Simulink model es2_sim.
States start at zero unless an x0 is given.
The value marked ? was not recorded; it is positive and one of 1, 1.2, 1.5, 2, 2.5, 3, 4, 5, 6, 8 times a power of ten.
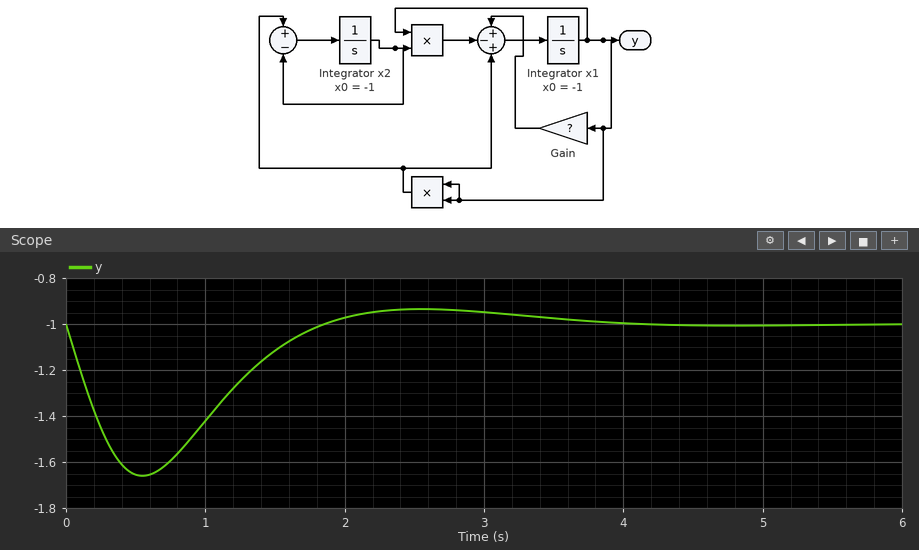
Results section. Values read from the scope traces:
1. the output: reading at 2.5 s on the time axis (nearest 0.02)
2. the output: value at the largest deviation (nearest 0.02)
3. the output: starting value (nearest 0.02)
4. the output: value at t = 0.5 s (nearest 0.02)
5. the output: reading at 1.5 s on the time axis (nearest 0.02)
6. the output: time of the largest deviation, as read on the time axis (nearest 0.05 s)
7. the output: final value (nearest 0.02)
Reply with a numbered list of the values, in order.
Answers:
1. -0.94
2. -1.66
3. -1.00
4. -1.66
5. -1.12
6. 0.55 s
7. -1.00
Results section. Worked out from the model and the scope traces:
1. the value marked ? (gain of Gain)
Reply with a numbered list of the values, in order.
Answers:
1. 2
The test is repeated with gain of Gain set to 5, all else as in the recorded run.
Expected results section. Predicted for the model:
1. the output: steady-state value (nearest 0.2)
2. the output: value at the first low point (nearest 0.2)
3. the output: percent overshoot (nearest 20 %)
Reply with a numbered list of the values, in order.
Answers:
1. -1.8
2. -3.2
3. 180 %
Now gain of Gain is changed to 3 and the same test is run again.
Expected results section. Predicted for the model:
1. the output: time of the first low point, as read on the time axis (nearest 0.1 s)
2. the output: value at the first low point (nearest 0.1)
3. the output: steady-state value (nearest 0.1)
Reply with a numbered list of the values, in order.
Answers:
1. 0.5 s
2. -2.2
3. -1.3
